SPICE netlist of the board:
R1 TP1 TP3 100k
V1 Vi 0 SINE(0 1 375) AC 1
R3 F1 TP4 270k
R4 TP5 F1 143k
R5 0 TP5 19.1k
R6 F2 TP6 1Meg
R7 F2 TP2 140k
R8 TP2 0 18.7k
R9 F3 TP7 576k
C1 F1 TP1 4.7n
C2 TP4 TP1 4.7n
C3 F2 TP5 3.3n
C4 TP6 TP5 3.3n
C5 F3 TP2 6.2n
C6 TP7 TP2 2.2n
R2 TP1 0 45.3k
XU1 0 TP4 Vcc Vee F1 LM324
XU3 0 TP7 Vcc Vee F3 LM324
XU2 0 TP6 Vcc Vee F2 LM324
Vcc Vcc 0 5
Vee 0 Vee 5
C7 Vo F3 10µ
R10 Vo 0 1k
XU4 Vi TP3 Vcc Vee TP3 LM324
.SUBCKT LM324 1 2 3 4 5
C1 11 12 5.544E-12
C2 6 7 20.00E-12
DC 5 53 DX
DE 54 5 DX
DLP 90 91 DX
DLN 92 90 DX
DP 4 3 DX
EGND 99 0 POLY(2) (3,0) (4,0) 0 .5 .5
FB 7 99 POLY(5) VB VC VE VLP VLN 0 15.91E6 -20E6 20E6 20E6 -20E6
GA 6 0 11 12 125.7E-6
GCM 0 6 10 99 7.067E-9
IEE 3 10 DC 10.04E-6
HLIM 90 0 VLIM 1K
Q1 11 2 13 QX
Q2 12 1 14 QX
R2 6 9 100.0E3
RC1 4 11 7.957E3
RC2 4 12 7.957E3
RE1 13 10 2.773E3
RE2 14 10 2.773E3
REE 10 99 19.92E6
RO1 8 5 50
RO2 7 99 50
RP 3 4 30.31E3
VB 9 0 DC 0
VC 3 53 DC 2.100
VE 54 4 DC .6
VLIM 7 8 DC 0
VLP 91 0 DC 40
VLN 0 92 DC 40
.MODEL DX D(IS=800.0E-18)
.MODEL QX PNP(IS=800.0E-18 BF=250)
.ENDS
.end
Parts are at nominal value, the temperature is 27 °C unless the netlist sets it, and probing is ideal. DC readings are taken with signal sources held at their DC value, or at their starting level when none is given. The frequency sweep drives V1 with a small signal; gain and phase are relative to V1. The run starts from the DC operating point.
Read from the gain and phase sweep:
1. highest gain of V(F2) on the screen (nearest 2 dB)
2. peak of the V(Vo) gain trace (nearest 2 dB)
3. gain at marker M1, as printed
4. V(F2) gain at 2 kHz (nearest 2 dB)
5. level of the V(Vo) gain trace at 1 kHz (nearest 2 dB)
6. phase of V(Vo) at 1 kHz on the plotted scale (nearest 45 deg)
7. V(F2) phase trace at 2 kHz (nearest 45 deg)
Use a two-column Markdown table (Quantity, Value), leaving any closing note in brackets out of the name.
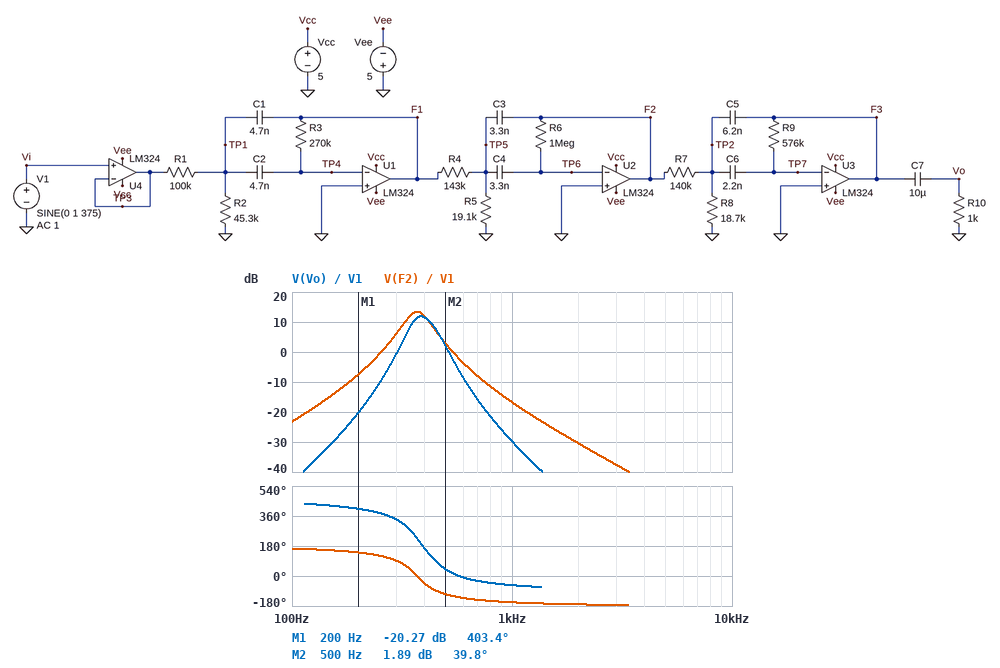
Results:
| Quantity | Value |
|---|---|
| highest gain of V(F2) on the screen | 14 dB |
| peak of the V(Vo) gain trace | 12 dB |
| gain at marker M1, as printed | -20.27 dB |
| V(F2) gain at 2 kHz | -30 dB |
| level of the V(Vo) gain trace at 1 kHz | -30 dB |
| phase of V(Vo) at 1 kHz on the plotted scale | -45 deg |
| V(F2) phase trace at 2 kHz | -180 deg |
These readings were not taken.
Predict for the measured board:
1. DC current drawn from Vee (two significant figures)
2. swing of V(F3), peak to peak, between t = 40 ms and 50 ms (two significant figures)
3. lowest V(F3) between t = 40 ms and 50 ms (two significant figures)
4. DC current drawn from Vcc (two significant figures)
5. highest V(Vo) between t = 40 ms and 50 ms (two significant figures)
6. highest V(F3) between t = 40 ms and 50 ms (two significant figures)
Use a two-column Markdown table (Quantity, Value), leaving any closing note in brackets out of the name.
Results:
| Quantity | Value |
|---|---|
| DC current drawn from Vee | 1.4 mA |
| swing of V(F3), peak to peak, between t = 40 ms and 50 ms | 6.3 V |
| lowest V(F3) between t = 40 ms and 50 ms | -3.2 V |
| DC current drawn from Vcc | 1.4 mA |
| highest V(Vo) between t = 40 ms and 50 ms | 3.1 V |
| highest V(F3) between t = 40 ms and 50 ms | 3.1 V |
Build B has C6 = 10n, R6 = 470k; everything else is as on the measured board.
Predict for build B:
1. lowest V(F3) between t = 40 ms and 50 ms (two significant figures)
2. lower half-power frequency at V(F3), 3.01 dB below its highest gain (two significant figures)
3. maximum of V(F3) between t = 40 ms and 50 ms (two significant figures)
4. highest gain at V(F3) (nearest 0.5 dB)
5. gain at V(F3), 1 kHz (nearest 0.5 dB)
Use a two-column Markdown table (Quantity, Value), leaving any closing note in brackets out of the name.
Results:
| Quantity | Value |
|---|---|
| lowest V(F3) between t = 40 ms and 50 ms | -690 mV |
| lower half-power frequency at V(F3), 3.01 dB below its highest gain | 210 Hz |
| maximum of V(F3) between t = 40 ms and 50 ms | 660 mV |
| highest gain at V(F3) | -3.0 dB |
| gain at V(F3), 1 kHz | -29.5 dB |
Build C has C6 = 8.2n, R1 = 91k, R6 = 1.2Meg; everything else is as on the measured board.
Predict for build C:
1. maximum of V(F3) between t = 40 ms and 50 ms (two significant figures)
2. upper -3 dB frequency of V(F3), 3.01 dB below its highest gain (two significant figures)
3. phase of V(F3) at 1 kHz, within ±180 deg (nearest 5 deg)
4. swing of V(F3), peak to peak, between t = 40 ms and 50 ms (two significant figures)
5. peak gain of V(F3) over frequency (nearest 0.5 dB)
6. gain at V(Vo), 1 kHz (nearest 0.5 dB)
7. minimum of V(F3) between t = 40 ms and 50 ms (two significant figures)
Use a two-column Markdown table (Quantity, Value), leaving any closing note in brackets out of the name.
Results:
| Quantity | Value |
|---|---|
| maximum of V(F3) between t = 40 ms and 50 ms | 2.9 V |
| upper -3 dB frequency of V(F3), 3.01 dB below its highest gain | 370 Hz |
| phase of V(F3) at 1 kHz, within ±180 deg | -65 deg |
| swing of V(F3), peak to peak, between t = 40 ms and 50 ms | 5.7 V |
| peak gain of V(F3) over frequency | 15.0 dB |
| gain at V(Vo), 1 kHz | -30.5 dB |
| minimum of V(F3) between t = 40 ms and 50 ms | -2.8 V |
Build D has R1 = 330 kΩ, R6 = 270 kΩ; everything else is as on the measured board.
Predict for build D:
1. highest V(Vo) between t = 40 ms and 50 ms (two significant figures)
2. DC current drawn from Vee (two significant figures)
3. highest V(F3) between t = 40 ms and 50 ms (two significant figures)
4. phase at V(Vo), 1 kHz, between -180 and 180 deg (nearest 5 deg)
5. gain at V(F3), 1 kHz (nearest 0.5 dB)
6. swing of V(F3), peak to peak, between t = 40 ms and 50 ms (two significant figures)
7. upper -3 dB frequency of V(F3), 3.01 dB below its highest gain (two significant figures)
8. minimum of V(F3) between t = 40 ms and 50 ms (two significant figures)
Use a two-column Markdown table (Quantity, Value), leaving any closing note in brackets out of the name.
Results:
| Quantity | Value |
|---|---|
| highest V(Vo) between t = 40 ms and 50 ms | 100 mV |
| DC current drawn from Vee | 1.4 mA |
| highest V(F3) between t = 40 ms and 50 ms | 90 mV |
| phase at V(Vo), 1 kHz, between -180 and 180 deg | -25 deg |
| gain at V(F3), 1 kHz | -37.5 dB |
| swing of V(F3), peak to peak, between t = 40 ms and 50 ms | 200 mV |
| upper -3 dB frequency of V(F3), 3.01 dB below its highest gain | 560 Hz |
| minimum of V(F3) between t = 40 ms and 50 ms | -110 mV |
